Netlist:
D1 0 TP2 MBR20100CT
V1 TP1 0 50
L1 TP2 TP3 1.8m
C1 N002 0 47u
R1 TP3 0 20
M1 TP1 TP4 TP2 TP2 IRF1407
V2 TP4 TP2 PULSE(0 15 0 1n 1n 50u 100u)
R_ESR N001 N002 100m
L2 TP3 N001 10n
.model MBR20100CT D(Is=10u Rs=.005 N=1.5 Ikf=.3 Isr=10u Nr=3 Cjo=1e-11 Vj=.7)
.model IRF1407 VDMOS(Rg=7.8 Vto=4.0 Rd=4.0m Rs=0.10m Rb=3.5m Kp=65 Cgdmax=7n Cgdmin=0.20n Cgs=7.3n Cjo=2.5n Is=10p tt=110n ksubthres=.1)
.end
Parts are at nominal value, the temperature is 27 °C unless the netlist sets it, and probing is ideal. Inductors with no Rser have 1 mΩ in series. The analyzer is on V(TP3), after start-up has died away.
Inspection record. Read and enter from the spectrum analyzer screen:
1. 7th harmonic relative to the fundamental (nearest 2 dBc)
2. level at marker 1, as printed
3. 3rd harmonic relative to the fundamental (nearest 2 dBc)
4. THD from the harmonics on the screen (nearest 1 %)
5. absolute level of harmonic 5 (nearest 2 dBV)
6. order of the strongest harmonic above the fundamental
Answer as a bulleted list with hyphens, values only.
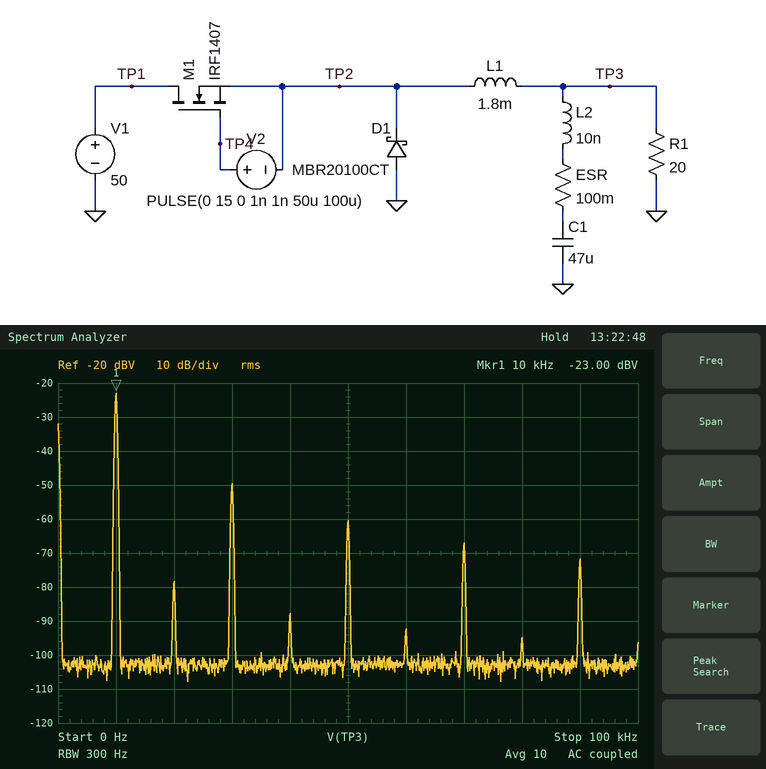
- -44 dBc
- -23.00 dBV
- -26 dBc
- 5 %
- -60 dBV
- 3
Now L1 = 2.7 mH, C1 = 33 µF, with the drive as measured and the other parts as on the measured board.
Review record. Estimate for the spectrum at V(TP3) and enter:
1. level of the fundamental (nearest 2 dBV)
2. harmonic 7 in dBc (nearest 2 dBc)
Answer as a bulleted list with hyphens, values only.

- -24 dBV
- -46 dBc
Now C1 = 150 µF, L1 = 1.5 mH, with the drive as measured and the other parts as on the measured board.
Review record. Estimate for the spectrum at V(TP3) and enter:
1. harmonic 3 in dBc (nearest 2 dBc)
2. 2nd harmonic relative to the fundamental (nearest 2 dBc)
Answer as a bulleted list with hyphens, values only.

- -22 dBc
- -52 dBc
